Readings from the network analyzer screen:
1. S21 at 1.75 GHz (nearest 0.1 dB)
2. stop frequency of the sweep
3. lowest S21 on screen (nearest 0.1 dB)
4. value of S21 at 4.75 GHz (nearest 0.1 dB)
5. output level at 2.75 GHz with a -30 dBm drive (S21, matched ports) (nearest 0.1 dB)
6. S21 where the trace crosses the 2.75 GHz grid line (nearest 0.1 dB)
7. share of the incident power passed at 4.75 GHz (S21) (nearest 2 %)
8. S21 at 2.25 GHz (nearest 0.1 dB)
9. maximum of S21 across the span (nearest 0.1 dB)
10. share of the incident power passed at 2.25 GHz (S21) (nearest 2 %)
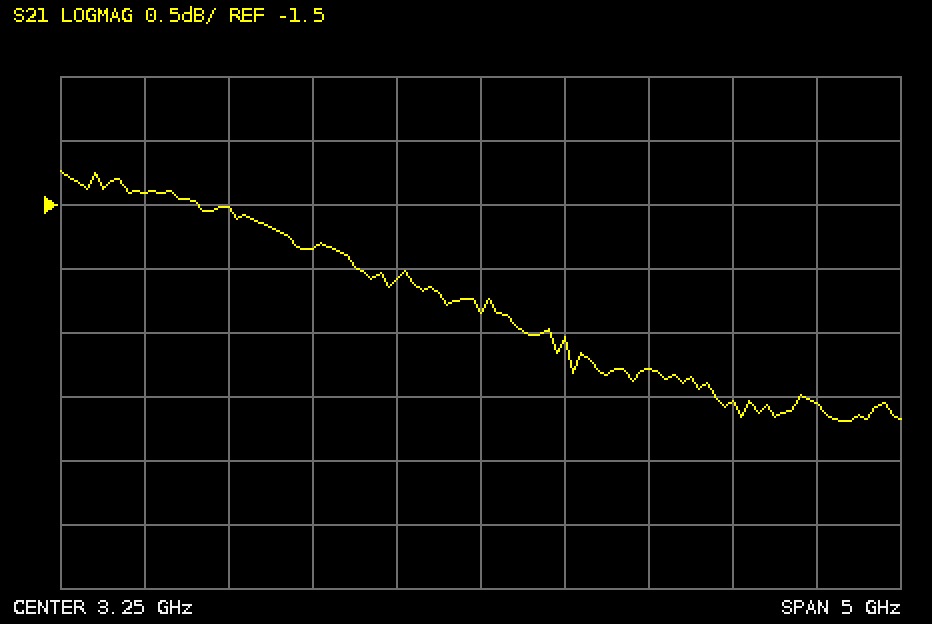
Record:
-1.5 dB
5.75 GHz
-3.2 dB
-3.0 dB
-32.1 dBm
-2.1 dB
50 %
-1.8 dB
-1.2 dB
66 %
